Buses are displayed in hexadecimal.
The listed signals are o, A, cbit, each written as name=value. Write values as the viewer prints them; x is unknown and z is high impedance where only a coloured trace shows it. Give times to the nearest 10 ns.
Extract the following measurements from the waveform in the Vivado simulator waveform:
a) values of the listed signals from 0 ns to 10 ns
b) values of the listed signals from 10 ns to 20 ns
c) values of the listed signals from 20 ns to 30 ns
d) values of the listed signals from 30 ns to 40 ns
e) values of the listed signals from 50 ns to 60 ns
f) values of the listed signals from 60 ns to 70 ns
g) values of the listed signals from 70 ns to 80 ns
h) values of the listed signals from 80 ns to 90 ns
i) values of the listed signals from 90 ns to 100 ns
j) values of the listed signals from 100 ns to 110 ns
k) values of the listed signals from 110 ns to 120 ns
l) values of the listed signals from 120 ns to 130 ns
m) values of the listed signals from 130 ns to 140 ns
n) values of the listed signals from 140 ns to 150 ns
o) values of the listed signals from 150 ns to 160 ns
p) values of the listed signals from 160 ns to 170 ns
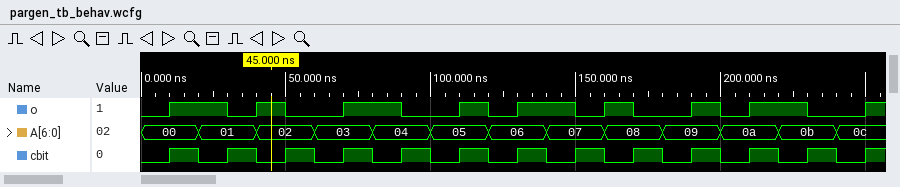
o=0, A=00, cbit=0
o=1, A=00, cbit=1
o=1, A=01, cbit=0
o=0, A=01, cbit=1
o=0, A=02, cbit=1
o=0, A=03, cbit=0
o=1, A=03, cbit=1
o=1, A=04, cbit=0
o=0, A=04, cbit=1
o=0, A=05, cbit=0
o=1, A=05, cbit=1
o=0, A=06, cbit=0
o=1, A=06, cbit=1
o=1, A=07, cbit=0
o=0, A=07, cbit=1
o=1, A=08, cbit=0
